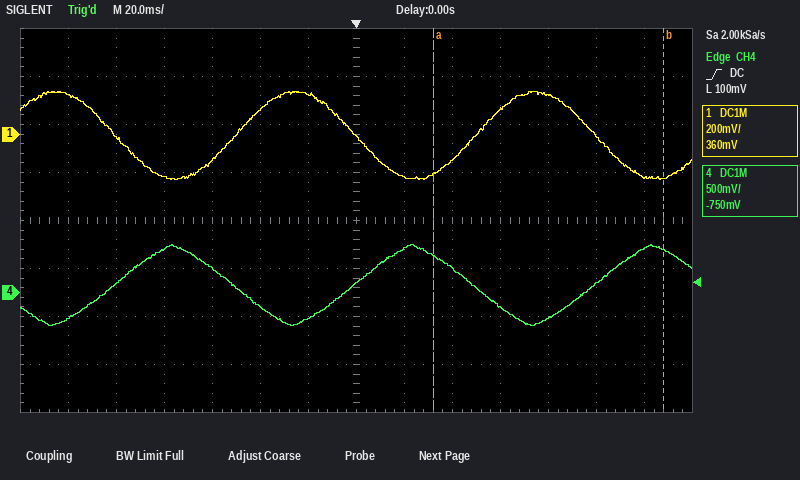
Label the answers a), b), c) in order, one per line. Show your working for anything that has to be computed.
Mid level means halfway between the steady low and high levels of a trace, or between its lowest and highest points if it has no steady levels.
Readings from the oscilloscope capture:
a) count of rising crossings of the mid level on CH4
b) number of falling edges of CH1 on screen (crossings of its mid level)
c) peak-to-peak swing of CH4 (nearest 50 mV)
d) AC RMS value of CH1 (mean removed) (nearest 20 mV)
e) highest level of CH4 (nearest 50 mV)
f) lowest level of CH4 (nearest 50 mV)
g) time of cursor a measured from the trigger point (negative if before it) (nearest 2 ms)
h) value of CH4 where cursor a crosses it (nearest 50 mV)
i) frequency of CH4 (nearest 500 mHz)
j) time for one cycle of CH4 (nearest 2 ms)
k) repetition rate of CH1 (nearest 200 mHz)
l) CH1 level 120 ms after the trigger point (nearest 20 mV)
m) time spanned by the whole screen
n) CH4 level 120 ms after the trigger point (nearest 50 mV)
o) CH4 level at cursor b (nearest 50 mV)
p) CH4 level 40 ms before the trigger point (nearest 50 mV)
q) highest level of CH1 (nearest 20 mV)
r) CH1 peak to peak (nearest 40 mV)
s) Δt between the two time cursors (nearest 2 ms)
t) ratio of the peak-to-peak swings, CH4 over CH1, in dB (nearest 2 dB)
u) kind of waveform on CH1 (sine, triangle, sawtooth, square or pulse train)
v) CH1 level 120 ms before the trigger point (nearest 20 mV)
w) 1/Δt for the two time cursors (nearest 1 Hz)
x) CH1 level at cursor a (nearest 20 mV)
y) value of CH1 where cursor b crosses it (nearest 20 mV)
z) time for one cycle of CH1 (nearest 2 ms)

a) 3
b) 3
c) 500 mV − (-350 mV) = 850 mV
d) 360 mV / (2√2) ≈ 127 mV, so 120 mV to the nearest 20 mV
e) 500 mV
f) -350 mV
g) +32 ms
h) 400 mV
i) 1 / 100 ms ≈ 10.0 Hz
j) 100 ms
k) 1 / 100 ms ≈ 10.0 Hz
l) -180 mV
m) 280 ms
n) 450 mV
o) 450 mV
p) -150 mV
q) 180 mV
r) 360 mV
s) 96 ms
t) 20 log10(850 mV / 360 mV) ≈ 7.46 dB, so 8 dB to the nearest 2 dB
u) sine
v) 160 mV
w) 1 / 96 ms ≈ 10 Hz
x) -160 mV
y) -180 mV
z) 100 ms
